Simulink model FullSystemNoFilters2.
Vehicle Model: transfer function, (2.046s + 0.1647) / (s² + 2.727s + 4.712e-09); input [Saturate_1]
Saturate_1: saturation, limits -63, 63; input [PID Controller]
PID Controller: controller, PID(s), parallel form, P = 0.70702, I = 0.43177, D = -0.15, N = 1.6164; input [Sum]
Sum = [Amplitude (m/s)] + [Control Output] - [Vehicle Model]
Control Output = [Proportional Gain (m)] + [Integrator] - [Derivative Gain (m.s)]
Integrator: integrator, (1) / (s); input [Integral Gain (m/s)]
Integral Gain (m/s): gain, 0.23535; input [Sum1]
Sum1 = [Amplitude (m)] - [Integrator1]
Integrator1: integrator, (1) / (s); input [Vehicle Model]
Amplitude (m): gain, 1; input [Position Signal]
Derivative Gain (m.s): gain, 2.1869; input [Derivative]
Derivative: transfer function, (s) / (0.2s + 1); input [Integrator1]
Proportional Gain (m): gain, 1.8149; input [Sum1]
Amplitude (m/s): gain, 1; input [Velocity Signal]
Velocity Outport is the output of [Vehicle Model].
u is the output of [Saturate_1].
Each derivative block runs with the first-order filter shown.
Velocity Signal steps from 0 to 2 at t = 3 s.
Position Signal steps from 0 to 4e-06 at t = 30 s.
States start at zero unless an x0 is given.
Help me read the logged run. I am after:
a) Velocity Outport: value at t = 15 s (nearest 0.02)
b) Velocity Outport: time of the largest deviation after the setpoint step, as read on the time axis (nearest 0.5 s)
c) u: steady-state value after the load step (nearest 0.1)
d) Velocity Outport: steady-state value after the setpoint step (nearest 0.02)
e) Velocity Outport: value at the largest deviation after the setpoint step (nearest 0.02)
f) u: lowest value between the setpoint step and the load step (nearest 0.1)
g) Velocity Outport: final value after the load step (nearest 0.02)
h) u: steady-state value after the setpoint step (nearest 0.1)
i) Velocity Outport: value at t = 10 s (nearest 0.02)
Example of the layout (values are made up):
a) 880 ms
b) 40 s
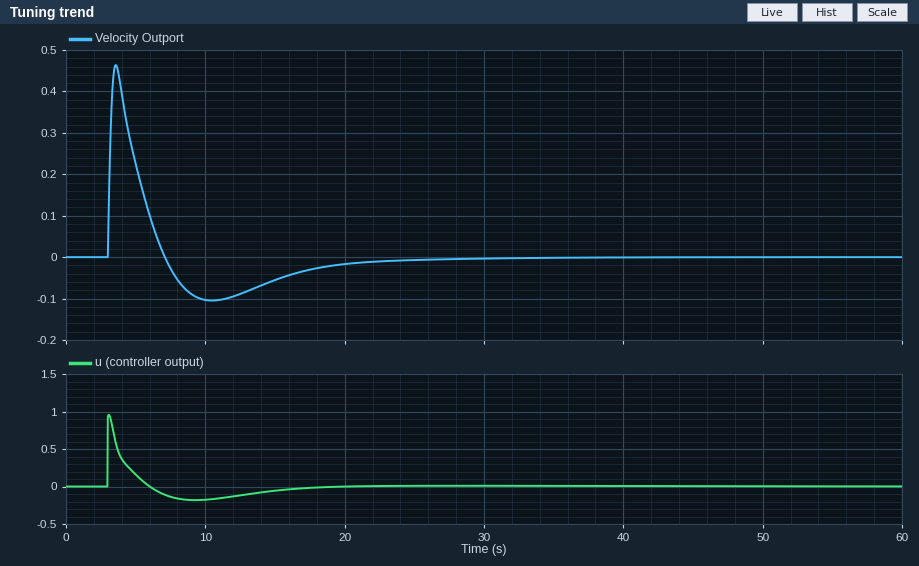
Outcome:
a) -0.06
b) 3.5 s
c) 0.0
d) 0.00
e) 0.46
f) -0.2
g) 0.00
h) 0.0
i) -0.10
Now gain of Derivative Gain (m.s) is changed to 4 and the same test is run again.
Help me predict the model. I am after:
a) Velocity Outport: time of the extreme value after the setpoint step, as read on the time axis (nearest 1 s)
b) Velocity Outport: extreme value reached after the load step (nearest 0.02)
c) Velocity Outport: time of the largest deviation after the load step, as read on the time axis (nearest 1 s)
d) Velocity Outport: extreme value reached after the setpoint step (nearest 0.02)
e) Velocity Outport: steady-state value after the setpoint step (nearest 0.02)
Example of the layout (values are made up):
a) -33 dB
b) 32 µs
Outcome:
a) 3 s
b) 0.00
c) 38 s
d) 0.38
e) 0.00
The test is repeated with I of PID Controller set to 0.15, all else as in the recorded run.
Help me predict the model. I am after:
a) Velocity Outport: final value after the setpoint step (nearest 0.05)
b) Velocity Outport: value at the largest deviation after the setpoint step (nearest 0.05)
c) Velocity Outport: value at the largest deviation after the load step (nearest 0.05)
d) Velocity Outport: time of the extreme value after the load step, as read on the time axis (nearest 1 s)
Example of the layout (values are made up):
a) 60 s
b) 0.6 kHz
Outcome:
a) 0.00
b) 0.40
c) 0.00
d) 36 s
